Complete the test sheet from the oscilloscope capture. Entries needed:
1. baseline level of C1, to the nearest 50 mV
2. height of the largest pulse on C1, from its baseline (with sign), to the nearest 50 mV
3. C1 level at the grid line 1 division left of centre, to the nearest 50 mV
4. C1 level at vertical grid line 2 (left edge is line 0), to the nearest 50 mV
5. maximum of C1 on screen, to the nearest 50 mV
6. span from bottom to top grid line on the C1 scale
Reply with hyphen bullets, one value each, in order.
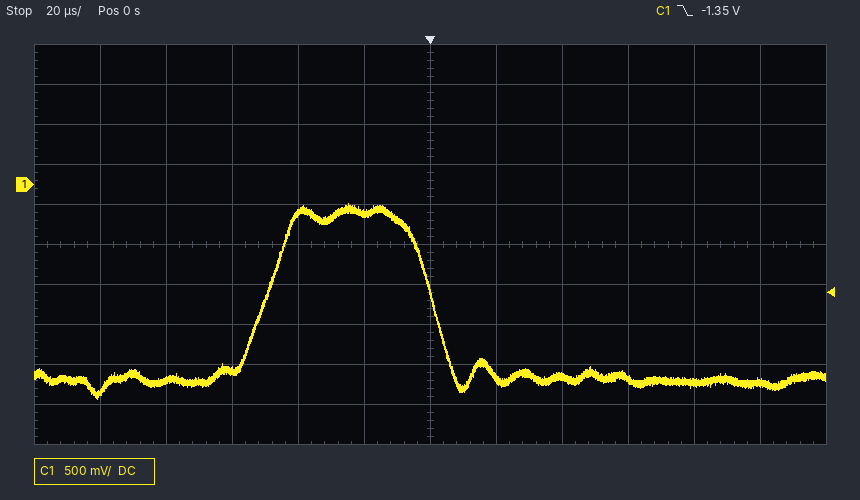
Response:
- -2.45 V
- +2.20 V
- -350 mV
- -2.45 V
- -250 mV
- 5 V
